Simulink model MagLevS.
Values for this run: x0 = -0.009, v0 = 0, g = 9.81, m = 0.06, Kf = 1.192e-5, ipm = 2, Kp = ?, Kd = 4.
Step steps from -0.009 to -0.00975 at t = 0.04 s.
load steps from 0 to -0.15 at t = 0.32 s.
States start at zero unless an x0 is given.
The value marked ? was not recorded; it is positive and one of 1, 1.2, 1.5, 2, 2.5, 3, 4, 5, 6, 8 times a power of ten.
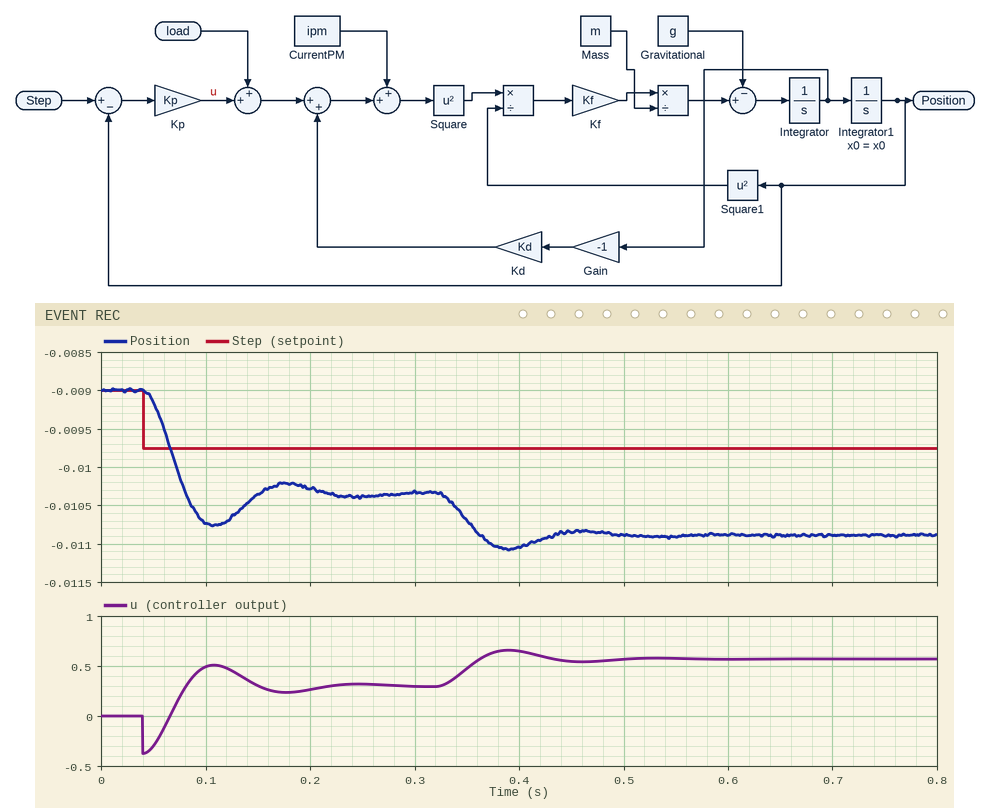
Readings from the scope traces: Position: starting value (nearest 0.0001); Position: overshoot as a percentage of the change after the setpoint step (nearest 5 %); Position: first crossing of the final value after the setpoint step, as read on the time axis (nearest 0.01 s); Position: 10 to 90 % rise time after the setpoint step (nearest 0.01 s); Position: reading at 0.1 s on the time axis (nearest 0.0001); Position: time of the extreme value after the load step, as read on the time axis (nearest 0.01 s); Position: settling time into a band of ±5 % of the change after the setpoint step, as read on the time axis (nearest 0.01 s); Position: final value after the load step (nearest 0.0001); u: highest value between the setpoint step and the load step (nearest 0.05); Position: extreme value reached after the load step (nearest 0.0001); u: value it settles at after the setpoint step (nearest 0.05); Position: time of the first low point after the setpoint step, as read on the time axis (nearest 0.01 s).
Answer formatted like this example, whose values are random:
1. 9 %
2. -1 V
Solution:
1. -0.0090
2. 30 %
3. 0.08 s
4. 0.03 s
5. -0.0107
6. 0.39 s
7. 0.20 s
8. -0.0109
9. 0.50
10. -0.0111
11. 0.30
12. 0.11 s
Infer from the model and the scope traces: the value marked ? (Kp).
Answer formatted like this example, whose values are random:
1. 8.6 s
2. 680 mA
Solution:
1. 500
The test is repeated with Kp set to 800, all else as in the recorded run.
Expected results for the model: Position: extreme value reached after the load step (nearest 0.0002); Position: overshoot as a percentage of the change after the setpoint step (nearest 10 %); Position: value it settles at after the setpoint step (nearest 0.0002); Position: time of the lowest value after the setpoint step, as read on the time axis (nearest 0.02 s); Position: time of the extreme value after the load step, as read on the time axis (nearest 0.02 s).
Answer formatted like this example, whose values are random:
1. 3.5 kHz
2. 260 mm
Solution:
1. -0.0104
2. 40 %
3. -0.0100
4. 0.08 s
5. 0.36 s
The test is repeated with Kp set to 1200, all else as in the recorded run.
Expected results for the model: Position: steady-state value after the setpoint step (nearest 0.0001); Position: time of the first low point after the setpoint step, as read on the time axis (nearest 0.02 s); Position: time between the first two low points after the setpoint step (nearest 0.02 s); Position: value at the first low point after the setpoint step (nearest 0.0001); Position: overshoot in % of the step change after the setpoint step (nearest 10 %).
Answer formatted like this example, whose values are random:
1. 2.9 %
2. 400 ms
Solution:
1. -0.0099
2. 0.08 s
3. 0.06 s
4. -0.0104
5. 50 %
